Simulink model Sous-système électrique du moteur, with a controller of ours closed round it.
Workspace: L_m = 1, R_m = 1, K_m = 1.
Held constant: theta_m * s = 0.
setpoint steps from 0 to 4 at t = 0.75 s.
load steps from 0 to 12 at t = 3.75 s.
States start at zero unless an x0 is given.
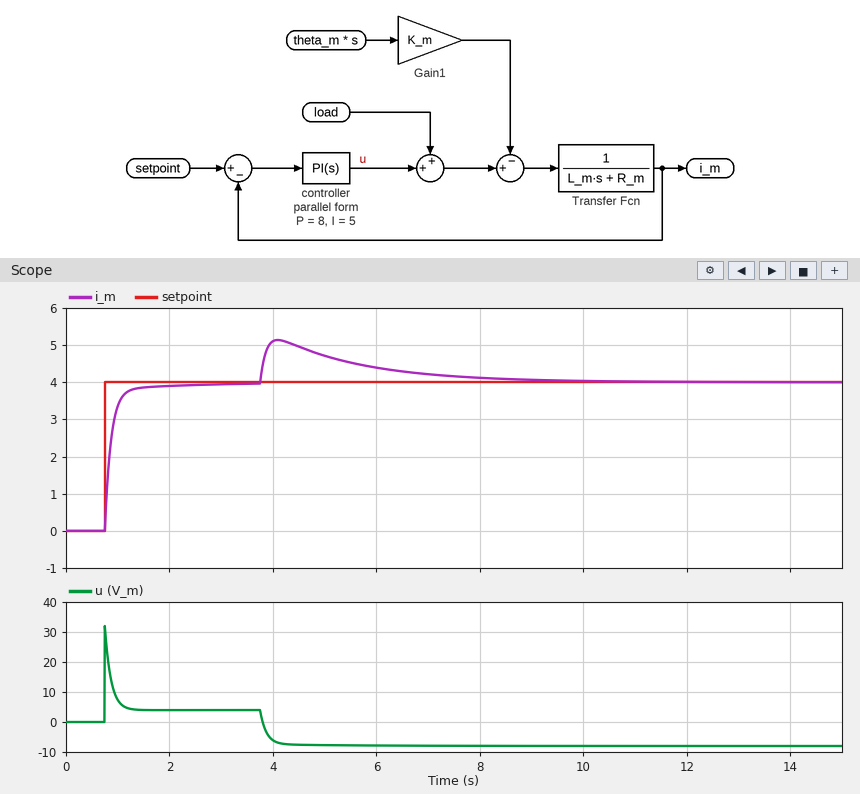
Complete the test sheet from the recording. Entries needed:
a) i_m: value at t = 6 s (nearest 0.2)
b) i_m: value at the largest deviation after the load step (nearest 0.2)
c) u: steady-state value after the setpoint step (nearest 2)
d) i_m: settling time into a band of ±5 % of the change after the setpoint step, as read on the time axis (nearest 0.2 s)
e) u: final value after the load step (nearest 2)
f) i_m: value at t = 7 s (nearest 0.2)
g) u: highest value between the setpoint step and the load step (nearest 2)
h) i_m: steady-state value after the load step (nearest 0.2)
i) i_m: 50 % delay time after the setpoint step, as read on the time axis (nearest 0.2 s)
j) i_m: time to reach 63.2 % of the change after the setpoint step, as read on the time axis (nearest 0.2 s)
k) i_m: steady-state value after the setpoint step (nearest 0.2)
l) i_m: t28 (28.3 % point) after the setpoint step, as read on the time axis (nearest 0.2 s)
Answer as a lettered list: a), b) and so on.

a) 4.4
b) 5.2
c) 4
d) 1.2 s
e) -8
f) 4.2
g) 32
h) 4.0
i) 0.8 s
j) 0.8 s
k) 4.0
l) 0.8 s
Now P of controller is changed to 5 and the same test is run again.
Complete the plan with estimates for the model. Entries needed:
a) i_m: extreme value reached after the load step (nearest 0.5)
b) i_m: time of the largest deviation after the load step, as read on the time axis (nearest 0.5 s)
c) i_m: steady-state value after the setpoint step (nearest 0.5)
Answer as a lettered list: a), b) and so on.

a) 5.5
b) 4.0 s
c) 4.0
